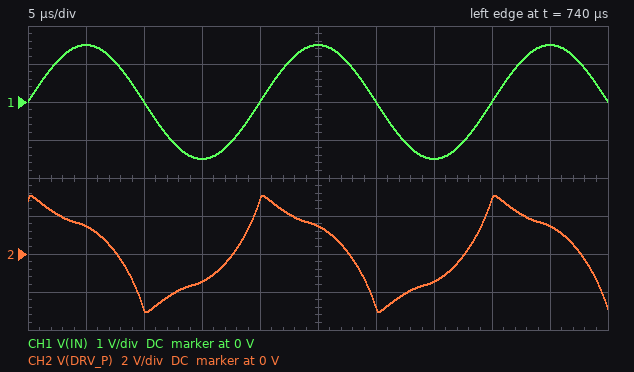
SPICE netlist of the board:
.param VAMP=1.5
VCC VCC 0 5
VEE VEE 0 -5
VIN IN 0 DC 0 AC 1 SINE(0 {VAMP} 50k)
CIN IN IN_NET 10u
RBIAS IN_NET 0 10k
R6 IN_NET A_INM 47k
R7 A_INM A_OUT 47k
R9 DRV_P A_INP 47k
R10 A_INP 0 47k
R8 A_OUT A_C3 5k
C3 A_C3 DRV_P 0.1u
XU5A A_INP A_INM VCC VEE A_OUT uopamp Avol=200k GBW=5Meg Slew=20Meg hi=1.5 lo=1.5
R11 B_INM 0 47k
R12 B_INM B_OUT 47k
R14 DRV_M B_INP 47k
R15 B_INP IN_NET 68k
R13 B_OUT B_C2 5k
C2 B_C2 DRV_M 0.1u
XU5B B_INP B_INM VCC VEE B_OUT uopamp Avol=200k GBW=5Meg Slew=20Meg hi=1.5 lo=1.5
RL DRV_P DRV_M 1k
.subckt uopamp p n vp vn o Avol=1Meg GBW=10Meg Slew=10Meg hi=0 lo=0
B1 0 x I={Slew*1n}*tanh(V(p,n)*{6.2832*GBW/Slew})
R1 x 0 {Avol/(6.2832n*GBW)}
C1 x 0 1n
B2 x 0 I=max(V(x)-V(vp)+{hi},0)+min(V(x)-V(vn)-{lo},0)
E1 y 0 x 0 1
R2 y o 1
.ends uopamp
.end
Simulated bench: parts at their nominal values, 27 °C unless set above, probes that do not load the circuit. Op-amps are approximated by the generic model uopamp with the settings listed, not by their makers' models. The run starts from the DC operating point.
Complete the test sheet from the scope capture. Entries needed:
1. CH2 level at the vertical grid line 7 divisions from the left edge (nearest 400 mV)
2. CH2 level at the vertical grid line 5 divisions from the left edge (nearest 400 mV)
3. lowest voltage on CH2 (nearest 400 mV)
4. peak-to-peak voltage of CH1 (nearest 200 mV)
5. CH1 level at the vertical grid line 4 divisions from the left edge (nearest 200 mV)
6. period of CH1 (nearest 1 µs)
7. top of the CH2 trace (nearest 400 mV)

-1.6 V
1.6 V
-3.2 V
3.0 V
0 V
20 µs
3.2 V
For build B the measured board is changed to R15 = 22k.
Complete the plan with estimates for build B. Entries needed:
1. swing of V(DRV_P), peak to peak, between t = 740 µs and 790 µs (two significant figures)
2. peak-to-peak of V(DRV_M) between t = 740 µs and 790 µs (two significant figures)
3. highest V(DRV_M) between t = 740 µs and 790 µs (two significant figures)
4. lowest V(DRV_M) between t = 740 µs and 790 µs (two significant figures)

2.1 V
2.7 V
1.4 V
-1.4 V
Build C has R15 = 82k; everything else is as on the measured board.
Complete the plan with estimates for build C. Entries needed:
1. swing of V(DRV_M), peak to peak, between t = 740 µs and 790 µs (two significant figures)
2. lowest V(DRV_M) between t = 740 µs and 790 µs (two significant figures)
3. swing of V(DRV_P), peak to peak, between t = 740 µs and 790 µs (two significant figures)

1.5 V
1.9 V
1.8 V
